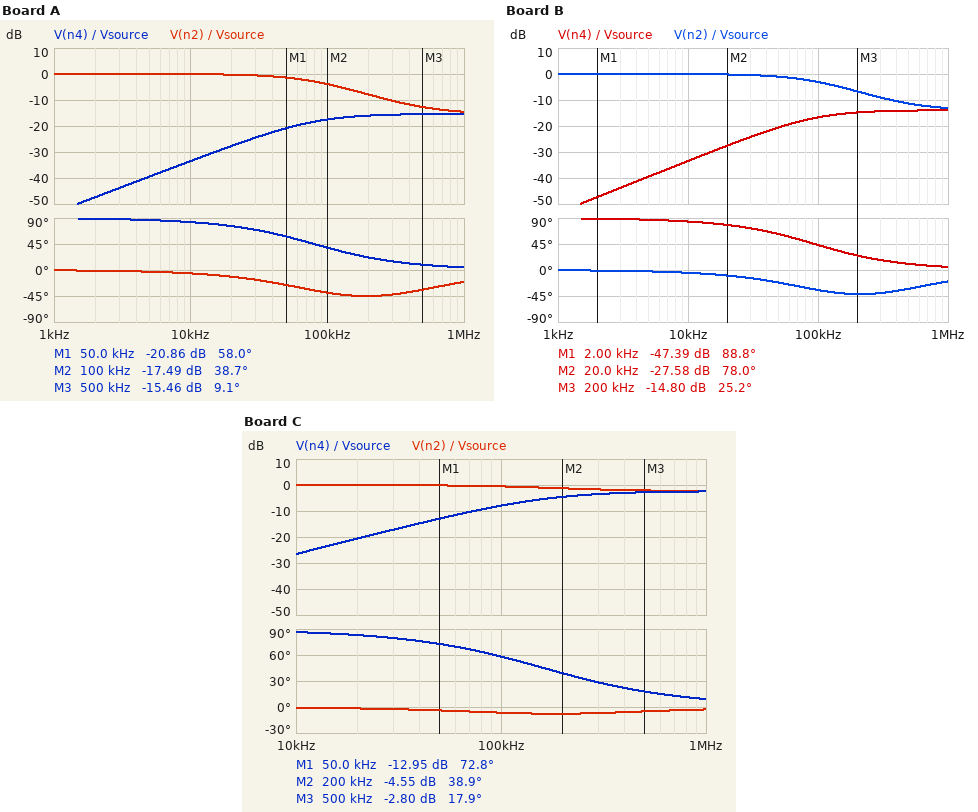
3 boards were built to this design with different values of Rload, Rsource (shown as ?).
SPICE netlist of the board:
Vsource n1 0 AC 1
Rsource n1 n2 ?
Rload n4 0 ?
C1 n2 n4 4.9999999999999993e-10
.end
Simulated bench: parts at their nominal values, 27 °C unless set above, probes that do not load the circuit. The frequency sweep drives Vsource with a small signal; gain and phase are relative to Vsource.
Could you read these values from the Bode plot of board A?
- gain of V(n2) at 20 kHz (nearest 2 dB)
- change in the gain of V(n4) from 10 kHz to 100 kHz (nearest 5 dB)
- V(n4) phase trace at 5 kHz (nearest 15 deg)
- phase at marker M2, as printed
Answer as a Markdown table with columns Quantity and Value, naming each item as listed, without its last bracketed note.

| Quantity | Value |
|---|---|
| gain of V(n2) at 20 kHz | 0 dB |
| change in the gain of V(n4) from 10 kHz to 100 kHz | 15 dB |
| V(n4) phase trace at 5 kHz | 90 deg |
| phase at marker M2, as printed | 38.7 deg |
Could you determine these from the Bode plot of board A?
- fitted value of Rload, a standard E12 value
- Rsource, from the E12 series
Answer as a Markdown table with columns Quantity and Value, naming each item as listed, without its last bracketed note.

| Quantity | Value |
|---|---|
| fitted value of Rload, a standard E12 value | 680 Ω |
| Rsource, from the E12 series | 3.3 kΩ |
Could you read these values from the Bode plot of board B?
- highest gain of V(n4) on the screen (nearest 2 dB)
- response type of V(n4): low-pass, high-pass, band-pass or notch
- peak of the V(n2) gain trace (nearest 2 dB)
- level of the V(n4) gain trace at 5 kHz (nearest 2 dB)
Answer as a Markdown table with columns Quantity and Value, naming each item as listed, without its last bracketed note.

| Quantity | Value |
|---|---|
| highest gain of V(n4) on the screen | -14 dB |
| response type of V(n4): low-pass, high-pass, band-pass or notch | high-pass |
| peak of the V(n2) gain trace | 0 dB |
| level of the V(n4) gain trace at 5 kHz | -40 dB |
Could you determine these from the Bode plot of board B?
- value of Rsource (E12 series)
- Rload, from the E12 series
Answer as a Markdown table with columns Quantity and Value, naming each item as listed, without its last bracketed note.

| Quantity | Value |
|---|---|
| value of Rsource | 2.7 kΩ |
| Rload, from the E12 series | 680 Ω |
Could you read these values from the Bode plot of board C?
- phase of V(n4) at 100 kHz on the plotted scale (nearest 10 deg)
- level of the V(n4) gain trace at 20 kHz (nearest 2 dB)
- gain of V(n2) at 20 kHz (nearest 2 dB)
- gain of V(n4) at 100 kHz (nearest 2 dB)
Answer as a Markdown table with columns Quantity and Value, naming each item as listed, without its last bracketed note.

| Quantity | Value |
|---|---|
| phase of V(n4) at 100 kHz on the plotted scale | 60 deg |
| level of the V(n4) gain trace at 20 kHz | -20 dB |
| gain of V(n2) at 20 kHz | 0 dB |
| gain of V(n4) at 100 kHz | -8 dB |
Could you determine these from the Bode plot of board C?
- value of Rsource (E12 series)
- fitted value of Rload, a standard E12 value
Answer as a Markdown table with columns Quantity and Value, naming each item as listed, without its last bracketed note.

| Quantity | Value |
|---|---|
| value of Rsource | 470 Ω |
| fitted value of Rload, a standard E12 value | 1.5 kΩ |
